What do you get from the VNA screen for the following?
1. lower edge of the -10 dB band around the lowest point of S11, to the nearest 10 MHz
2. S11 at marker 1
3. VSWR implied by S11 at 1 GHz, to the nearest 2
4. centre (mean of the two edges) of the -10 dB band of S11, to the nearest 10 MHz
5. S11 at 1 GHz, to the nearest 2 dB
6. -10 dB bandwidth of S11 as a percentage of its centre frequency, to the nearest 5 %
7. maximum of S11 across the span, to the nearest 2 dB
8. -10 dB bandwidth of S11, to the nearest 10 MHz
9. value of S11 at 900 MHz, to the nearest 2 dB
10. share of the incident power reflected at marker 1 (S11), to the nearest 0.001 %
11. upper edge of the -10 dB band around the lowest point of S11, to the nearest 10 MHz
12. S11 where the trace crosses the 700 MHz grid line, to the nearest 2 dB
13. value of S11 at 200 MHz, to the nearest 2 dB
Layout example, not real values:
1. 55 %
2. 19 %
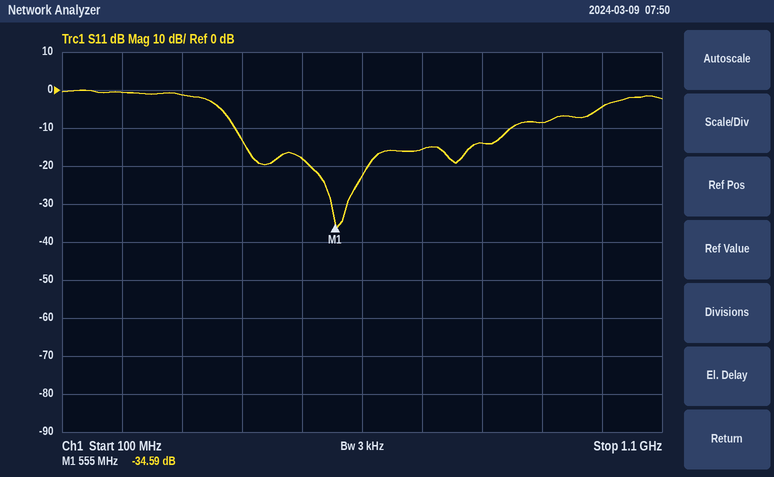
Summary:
1. 390 MHz
2. -34.59 dB
3. 4
4. 620 MHz
5. -4 dB
6. 75 %
7. 0 dB
8. 460 MHz
9. -8 dB
10. 0.035 %
11. 850 MHz
12. -16 dB
13. 0 dB
